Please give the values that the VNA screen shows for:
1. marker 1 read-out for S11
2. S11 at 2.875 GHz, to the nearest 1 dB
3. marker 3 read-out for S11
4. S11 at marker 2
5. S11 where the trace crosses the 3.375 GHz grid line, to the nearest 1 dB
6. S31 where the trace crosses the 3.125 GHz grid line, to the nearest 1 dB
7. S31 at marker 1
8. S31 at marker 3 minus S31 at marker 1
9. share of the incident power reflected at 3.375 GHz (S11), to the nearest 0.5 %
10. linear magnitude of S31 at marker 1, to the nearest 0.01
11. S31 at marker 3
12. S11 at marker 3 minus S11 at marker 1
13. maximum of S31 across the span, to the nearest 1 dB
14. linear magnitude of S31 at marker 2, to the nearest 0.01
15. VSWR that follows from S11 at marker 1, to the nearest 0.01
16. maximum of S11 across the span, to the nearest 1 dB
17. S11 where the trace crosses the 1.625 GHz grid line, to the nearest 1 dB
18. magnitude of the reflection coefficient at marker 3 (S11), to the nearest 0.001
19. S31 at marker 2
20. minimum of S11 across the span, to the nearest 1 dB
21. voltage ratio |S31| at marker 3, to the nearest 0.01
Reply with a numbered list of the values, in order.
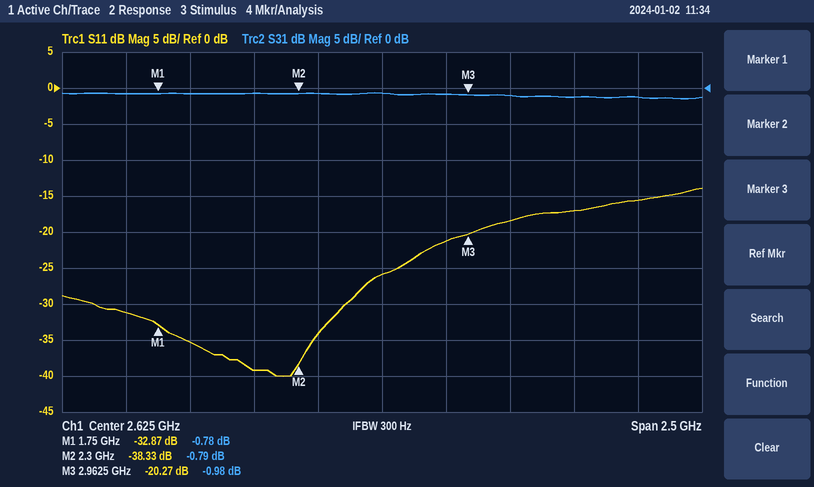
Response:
1. -32.87 dB
2. -21 dB
3. -20.27 dB
4. -38.33 dB
5. -17 dB
6. -1 dB
7. -0.78 dB
8. -0.20 dB
9. 2.0 %
10. 0.91
11. -0.98 dB
12. 12.60 dB
13. -1 dB
14. 0.91
15. 1.05
16. -14 dB
17. -31 dB
18. 0.097
19. -0.79 dB
20. -40 dB
21. 0.89
